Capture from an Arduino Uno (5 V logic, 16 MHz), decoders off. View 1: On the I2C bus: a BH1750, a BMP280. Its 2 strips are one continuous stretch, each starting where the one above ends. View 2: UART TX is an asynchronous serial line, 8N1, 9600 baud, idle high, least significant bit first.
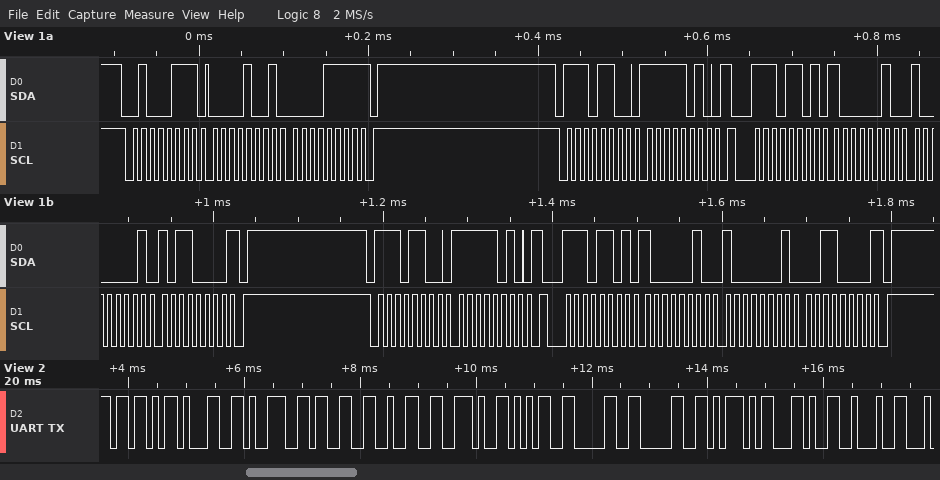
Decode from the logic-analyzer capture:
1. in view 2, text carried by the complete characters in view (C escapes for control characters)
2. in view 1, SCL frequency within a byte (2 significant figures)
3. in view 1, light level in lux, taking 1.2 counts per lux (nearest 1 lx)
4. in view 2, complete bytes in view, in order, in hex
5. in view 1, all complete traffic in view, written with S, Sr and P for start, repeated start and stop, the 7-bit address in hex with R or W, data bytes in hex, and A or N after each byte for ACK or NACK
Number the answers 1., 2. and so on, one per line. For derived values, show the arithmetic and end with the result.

1. "[1932.500],\""
2. 100 kHz
3. 2319 / 1.2 = 1932 lx
4. 5B 31 39 33 32 2E 35 30 30 5D 2C 22
5. S 23R A 09 A 0F N P S 76W A FA A Sr 76R A 82 A 81 A B0 N P S 76W A FA A Sr 76R A 82 A 81 A 30 N P
